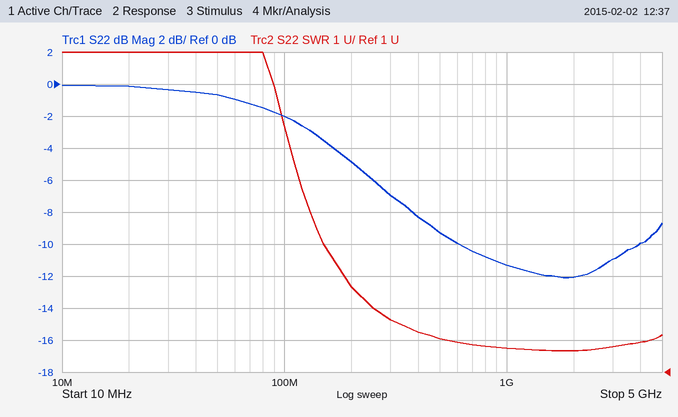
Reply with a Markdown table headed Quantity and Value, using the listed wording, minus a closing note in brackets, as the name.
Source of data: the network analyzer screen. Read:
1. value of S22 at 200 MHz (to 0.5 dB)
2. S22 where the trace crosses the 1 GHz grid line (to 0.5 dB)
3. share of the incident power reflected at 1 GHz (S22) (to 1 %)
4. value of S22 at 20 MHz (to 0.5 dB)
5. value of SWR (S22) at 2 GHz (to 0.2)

| Quantity | Value |
|---|---|
| value of S22 at 200 MHz | -5.0 dB |
| S22 where the trace crosses the 1 GHz grid line | -11.5 dB |
| share of the incident power reflected at 1 GHz (S22) | 7 % |
| value of S22 at 20 MHz | 0.0 dB |
| value of SWR (S22) at 2 GHz | 1.6 |
